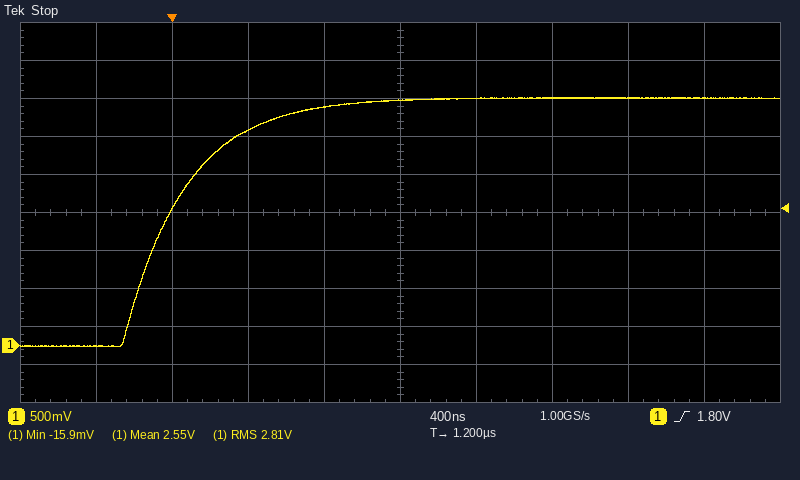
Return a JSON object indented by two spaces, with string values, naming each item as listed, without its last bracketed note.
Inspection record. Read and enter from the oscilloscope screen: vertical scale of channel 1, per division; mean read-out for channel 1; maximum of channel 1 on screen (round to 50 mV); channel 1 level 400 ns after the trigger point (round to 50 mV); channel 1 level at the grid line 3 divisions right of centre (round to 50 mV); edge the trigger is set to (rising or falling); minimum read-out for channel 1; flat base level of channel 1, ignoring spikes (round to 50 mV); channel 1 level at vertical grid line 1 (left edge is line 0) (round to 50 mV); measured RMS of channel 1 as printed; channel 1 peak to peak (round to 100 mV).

{
  "vertical scale of channel 1, per division": "500 mV",
  "mean read-out for channel 1": "2.55 V",
  "maximum of channel 1 on screen": "3.25 V",
  "channel 1 level 400 ns after the trigger point": "2.85 V",
  "channel 1 level at the grid line 3 divisions right of centre": "3.25 V",
  "edge the trigger is set to": "rising",
  "minimum read-out for channel 1": "-15.9 mV",
  "flat base level of channel 1, ignoring spikes": "0 mV",
  "channel 1 level at vertical grid line 1 (left edge is line 0)": "0 mV",
  "measured RMS of channel 1 as printed": "2.81 V",
  "channel 1 peak to peak": "3.30 V"
}
